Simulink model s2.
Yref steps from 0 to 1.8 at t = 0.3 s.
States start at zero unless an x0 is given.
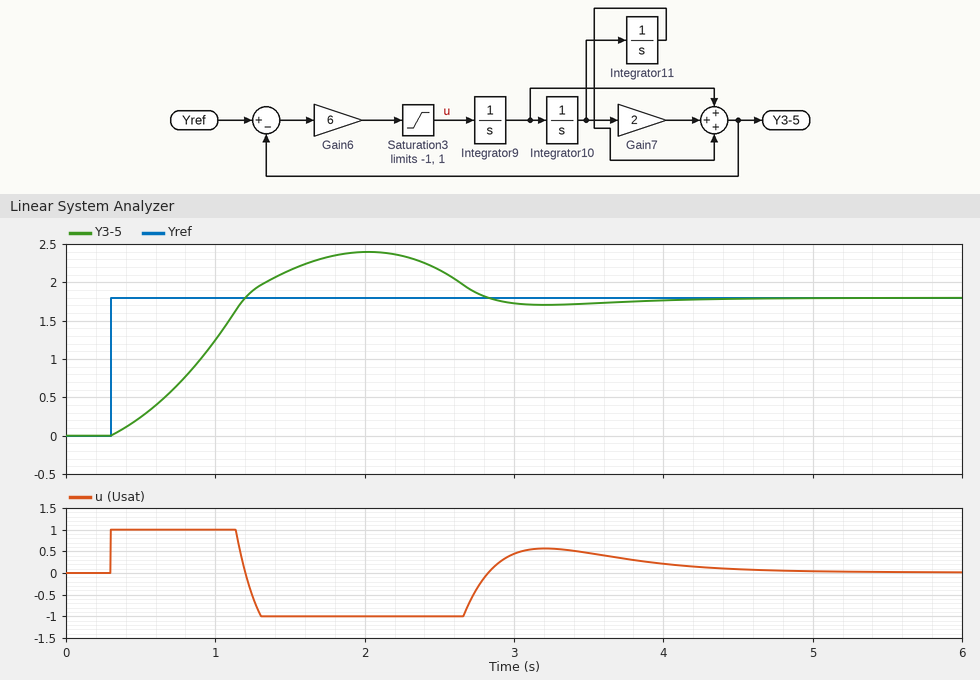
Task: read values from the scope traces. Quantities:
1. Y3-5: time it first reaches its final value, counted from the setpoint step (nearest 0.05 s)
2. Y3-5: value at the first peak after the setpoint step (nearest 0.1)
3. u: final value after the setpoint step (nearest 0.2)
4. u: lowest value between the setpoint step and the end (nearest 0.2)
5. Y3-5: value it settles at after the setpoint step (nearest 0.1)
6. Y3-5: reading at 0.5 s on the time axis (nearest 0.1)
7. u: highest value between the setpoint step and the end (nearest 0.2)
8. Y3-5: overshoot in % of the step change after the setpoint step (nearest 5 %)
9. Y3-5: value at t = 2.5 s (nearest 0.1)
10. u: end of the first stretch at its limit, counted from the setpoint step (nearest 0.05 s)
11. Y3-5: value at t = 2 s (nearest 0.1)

0.90 s
2.4
0.0
-1.0
1.8
0.2
1.0
35 %
2.2
0.85 s
2.4
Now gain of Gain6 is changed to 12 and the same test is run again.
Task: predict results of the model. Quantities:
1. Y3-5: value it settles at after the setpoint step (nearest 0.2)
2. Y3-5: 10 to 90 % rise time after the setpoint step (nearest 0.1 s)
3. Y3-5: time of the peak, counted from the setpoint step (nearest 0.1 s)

1.8
0.7 s
1.7 s
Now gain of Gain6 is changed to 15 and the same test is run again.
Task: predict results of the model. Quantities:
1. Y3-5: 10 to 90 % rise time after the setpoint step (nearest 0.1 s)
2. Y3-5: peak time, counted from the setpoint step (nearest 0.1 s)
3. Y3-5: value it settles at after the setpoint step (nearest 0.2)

0.7 s
1.7 s
1.8
